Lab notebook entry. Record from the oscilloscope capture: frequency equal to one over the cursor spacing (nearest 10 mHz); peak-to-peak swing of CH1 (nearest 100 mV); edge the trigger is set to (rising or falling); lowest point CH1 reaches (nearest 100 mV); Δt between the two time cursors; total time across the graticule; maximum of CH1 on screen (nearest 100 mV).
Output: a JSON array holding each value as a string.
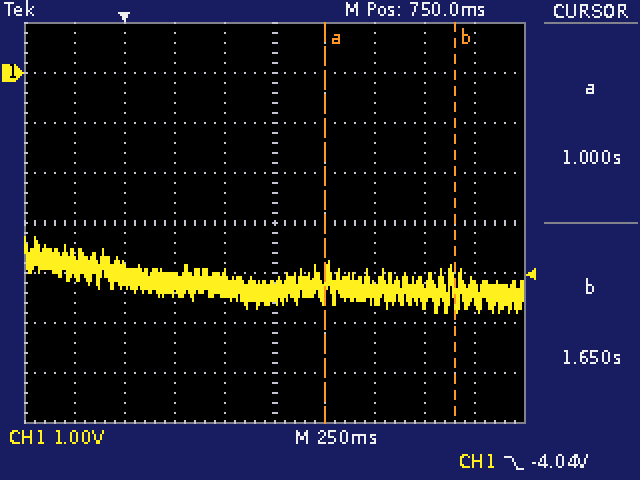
["1.54 Hz", "1.5 V", "falling", "-4.8 V", "650 ms", "2.5 s", "-3.3 V"]
